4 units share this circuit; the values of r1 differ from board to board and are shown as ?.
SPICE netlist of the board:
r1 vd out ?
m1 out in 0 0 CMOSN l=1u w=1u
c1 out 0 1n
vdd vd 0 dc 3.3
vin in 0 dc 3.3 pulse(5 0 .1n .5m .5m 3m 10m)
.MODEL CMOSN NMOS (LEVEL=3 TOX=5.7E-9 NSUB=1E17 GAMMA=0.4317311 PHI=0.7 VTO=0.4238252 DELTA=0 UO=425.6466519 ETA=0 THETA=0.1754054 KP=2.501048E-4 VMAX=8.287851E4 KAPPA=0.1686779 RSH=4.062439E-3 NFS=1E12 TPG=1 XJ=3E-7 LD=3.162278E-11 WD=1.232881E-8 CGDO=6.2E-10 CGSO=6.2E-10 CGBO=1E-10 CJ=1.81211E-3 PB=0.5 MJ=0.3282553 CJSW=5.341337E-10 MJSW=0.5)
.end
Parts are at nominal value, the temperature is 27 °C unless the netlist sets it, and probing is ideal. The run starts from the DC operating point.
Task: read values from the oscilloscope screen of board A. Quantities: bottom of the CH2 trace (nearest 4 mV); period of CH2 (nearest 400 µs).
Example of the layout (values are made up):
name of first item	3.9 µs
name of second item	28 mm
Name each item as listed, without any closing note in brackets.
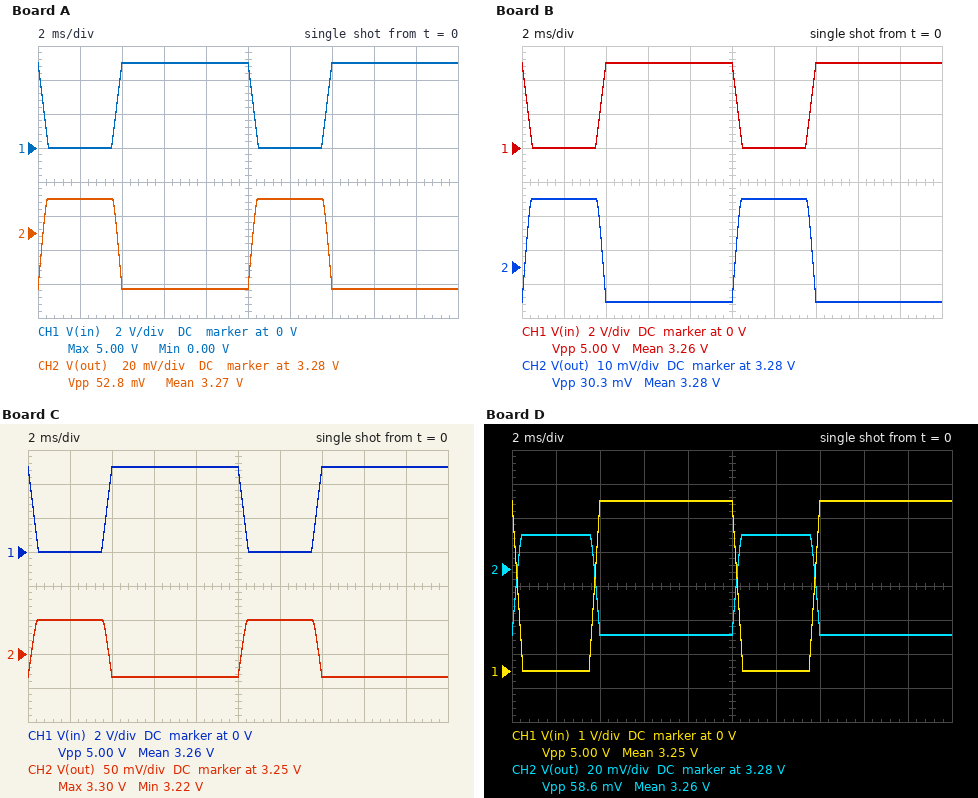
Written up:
bottom of the CH2 trace	3.248 V
period of CH2	10.0 ms
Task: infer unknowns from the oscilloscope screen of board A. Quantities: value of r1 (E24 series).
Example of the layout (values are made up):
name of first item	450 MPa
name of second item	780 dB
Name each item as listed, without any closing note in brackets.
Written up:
value of r1	82 Ω
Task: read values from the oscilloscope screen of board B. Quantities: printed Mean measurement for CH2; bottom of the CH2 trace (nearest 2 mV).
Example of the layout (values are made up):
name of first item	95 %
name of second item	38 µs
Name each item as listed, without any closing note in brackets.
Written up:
printed Mean measurement for CH2	3.28 V
bottom of the CH2 trace	3.270 V
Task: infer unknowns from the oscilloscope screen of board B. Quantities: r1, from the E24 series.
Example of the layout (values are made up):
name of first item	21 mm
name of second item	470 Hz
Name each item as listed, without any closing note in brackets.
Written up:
r1, from the E24 series	47 Ω
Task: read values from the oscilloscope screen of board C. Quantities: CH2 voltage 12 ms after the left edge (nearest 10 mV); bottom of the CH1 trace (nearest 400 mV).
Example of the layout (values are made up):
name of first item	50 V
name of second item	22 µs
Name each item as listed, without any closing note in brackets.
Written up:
CH2 voltage 12 ms after the left edge	3.30 V
bottom of the CH1 trace	0 V
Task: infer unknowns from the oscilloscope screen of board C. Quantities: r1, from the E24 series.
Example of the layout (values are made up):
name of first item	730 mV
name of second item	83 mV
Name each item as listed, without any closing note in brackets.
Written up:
r1, from the E24 series	130 Ω
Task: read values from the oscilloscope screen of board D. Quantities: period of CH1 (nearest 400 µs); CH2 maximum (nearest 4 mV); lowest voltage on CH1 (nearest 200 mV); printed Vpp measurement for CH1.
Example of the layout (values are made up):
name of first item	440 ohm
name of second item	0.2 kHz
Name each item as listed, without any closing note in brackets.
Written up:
period of CH1	10.0 ms
CH2 maximum	3.300 V
lowest voltage on CH1	0 V
printed Vpp measurement for CH1	5.00 V
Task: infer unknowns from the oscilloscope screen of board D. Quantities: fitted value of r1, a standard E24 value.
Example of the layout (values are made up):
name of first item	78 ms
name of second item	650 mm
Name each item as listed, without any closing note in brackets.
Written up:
fitted value of r1, a standard E24 value	91 Ω
